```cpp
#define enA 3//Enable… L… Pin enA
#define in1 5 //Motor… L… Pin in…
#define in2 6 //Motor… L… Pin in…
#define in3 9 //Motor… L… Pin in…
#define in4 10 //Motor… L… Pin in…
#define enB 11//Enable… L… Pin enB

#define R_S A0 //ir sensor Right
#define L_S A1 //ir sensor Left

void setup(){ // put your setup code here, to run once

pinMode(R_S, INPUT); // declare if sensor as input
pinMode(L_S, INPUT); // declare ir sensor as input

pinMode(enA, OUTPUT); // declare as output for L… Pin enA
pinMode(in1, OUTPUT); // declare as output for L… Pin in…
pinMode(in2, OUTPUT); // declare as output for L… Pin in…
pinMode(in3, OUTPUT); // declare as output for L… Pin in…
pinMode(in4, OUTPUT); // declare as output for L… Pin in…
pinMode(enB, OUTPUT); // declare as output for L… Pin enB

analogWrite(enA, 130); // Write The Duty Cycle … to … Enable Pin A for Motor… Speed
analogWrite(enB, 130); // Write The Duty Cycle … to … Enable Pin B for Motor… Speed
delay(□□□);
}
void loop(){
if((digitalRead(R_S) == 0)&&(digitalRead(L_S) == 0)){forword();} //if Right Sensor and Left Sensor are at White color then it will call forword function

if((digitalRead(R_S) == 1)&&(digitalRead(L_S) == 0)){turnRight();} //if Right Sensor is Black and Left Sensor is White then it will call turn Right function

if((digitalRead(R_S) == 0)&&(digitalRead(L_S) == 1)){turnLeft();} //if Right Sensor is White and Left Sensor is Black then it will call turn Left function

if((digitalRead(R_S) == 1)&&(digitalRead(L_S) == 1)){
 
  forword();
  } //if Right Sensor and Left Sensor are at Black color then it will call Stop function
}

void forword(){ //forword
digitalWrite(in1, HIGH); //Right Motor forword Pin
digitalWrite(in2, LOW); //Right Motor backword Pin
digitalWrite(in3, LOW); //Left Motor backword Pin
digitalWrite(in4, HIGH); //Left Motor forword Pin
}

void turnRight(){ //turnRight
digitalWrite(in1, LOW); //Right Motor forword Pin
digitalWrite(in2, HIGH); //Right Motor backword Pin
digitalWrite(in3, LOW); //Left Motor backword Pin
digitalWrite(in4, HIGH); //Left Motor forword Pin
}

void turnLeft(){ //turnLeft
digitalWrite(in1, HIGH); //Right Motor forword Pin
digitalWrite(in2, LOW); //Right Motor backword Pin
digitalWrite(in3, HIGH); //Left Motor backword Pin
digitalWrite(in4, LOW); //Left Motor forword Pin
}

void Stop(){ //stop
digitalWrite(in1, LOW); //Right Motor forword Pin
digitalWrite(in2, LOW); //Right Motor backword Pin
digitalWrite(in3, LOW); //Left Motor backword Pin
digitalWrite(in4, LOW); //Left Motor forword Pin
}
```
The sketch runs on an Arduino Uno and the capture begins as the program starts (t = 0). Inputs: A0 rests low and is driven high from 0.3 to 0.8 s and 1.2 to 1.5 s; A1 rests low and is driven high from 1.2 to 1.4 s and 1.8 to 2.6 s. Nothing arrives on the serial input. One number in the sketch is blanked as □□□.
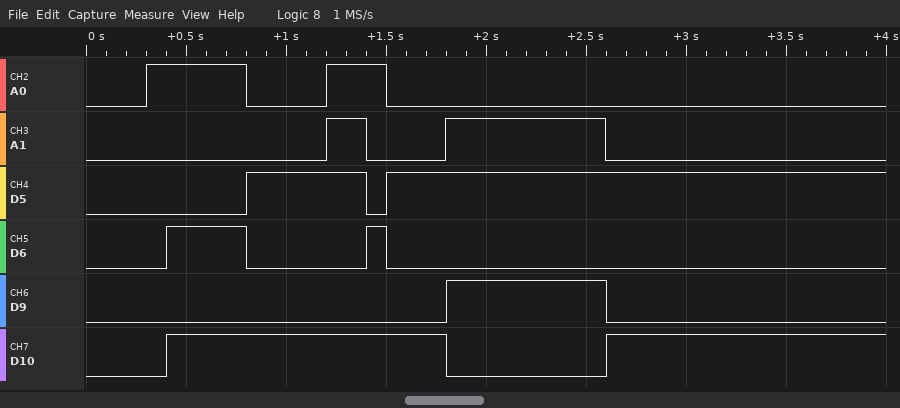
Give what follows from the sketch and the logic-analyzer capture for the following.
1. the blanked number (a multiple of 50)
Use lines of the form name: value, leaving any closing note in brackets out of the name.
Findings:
the blanked number: 400
